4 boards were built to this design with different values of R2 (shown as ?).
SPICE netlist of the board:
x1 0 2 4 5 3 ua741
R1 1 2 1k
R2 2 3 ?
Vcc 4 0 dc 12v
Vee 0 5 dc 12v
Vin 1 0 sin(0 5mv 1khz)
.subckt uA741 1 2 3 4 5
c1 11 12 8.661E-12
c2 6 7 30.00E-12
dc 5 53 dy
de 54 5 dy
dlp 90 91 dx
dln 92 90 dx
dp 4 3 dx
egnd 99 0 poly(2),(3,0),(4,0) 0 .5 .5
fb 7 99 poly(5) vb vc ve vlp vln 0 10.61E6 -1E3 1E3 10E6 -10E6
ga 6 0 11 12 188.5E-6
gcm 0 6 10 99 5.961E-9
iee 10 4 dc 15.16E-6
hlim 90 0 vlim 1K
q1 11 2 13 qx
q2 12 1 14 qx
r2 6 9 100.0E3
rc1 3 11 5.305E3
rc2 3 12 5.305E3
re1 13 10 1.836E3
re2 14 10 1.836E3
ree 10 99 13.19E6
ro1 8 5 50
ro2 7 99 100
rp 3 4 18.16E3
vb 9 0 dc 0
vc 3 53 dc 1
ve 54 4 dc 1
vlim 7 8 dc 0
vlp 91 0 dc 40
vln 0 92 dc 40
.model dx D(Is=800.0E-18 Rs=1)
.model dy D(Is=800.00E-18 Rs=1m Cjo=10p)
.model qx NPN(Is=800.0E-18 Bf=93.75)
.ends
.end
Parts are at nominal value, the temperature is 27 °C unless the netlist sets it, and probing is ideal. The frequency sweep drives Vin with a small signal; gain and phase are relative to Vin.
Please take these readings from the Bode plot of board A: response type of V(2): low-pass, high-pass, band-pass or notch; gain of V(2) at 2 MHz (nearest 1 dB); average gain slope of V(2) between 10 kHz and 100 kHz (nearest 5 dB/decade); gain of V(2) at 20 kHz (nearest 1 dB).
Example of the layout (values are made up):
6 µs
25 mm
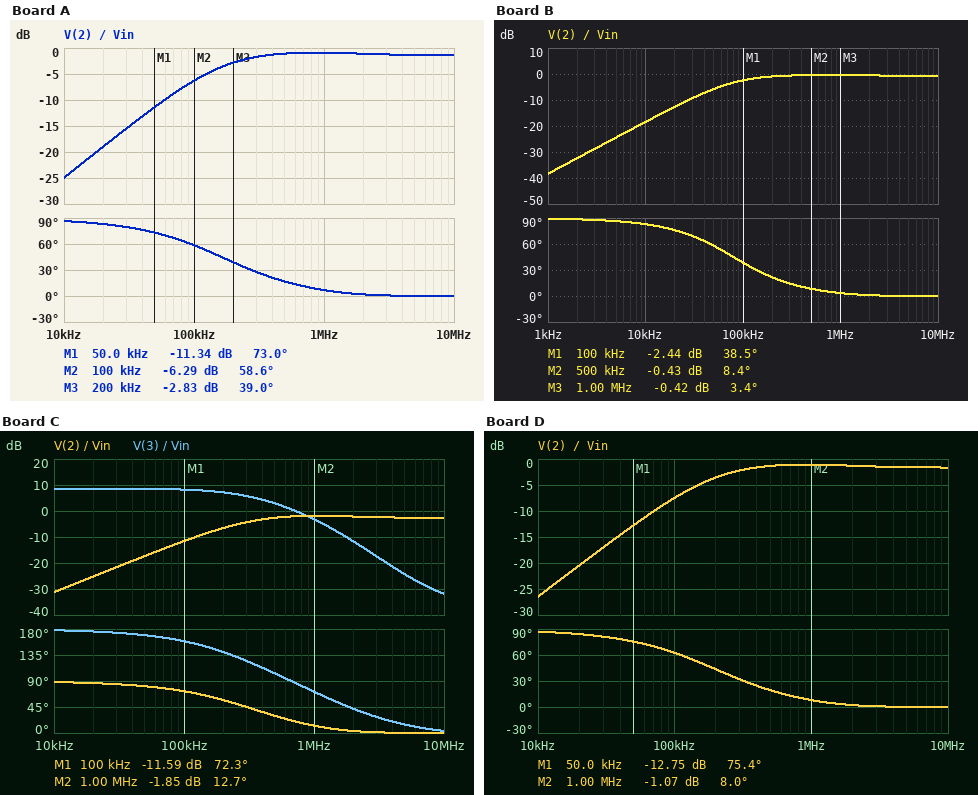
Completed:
high-pass
-1 dB
20 dB/decade
-19 dB
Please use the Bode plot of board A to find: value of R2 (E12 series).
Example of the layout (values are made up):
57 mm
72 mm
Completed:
5.6 kΩ
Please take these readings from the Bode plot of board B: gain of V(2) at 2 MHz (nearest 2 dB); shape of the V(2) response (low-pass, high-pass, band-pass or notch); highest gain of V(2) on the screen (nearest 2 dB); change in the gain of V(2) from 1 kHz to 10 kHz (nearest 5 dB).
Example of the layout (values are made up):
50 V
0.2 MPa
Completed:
0 dB
high-pass
0 dB
20 dB
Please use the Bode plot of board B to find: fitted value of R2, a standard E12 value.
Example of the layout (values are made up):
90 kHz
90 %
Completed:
12 kΩ
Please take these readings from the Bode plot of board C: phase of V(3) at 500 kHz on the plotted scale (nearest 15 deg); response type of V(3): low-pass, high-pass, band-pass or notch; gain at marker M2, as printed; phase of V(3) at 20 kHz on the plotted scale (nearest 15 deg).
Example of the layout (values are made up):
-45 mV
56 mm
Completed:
105 deg
low-pass
-1.85 dB
180 deg
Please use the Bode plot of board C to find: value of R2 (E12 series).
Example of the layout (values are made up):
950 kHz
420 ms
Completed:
2.7 kΩ
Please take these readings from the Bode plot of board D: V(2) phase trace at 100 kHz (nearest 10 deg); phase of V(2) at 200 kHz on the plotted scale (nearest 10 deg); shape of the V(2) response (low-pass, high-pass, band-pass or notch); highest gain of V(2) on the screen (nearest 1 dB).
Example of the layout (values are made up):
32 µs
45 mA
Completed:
60 deg
40 deg
high-pass
-1 dB
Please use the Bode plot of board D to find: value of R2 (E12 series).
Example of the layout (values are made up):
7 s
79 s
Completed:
4.7 kΩ
